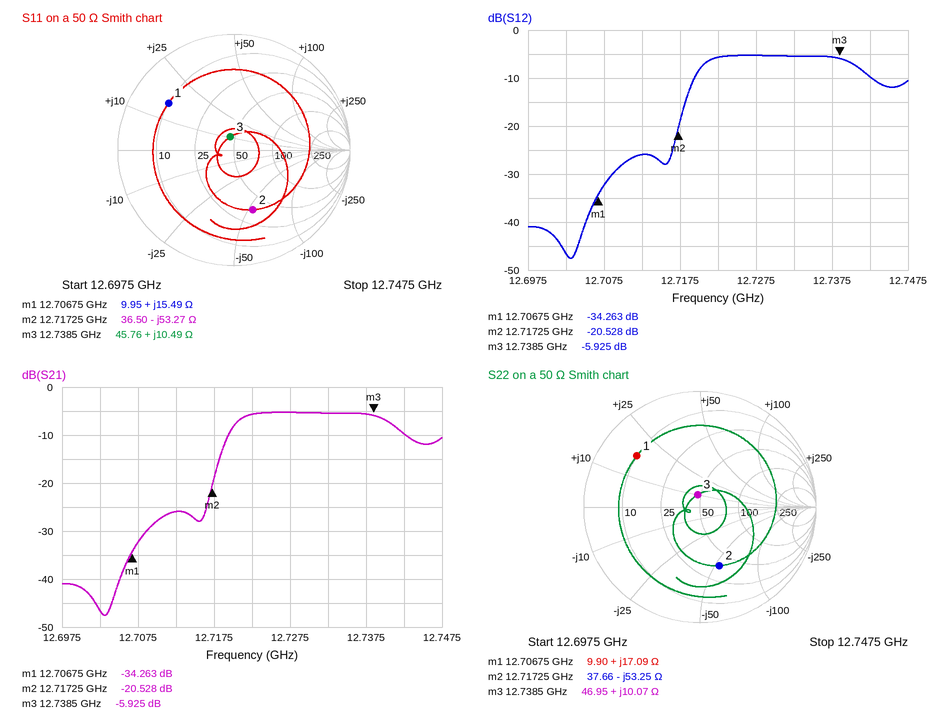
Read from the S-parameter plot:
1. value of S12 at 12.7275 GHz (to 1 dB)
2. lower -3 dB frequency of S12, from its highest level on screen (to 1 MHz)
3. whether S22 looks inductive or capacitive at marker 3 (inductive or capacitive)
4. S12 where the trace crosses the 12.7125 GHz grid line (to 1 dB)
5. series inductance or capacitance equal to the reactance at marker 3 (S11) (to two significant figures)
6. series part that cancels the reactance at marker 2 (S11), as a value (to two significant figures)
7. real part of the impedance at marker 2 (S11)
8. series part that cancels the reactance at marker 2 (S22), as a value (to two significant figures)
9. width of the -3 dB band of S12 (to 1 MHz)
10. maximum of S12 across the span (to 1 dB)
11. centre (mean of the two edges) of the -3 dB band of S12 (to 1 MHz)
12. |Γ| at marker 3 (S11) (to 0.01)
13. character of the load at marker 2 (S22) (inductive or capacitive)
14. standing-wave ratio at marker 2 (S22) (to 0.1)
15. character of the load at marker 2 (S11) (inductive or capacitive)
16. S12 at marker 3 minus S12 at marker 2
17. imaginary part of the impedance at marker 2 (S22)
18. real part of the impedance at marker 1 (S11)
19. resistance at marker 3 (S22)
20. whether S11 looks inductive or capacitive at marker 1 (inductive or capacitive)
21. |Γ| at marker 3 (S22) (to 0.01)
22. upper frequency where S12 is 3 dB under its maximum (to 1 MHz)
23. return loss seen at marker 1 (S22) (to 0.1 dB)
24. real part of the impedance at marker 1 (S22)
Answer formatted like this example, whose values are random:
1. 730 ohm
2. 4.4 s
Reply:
1. -5 dB
2. 12.720 GHz
3. inductive
4. -26 dB
5. 130 pH
6. 670 pH
7. 36.50 Ω
8. 670 pH
9. 21 MHz
10. -5 dB
11. 12.731 GHz
12. 0.12
13. capacitive
14. 3.3
15. capacitive
16. 14.603 dB
17. -53.25 Ω
18. 9.95 Ω
19. 46.95 Ω
20. inductive
21. 0.11
22. 12.741 GHz
23. 3.1 dB
24. 9.90 Ω
